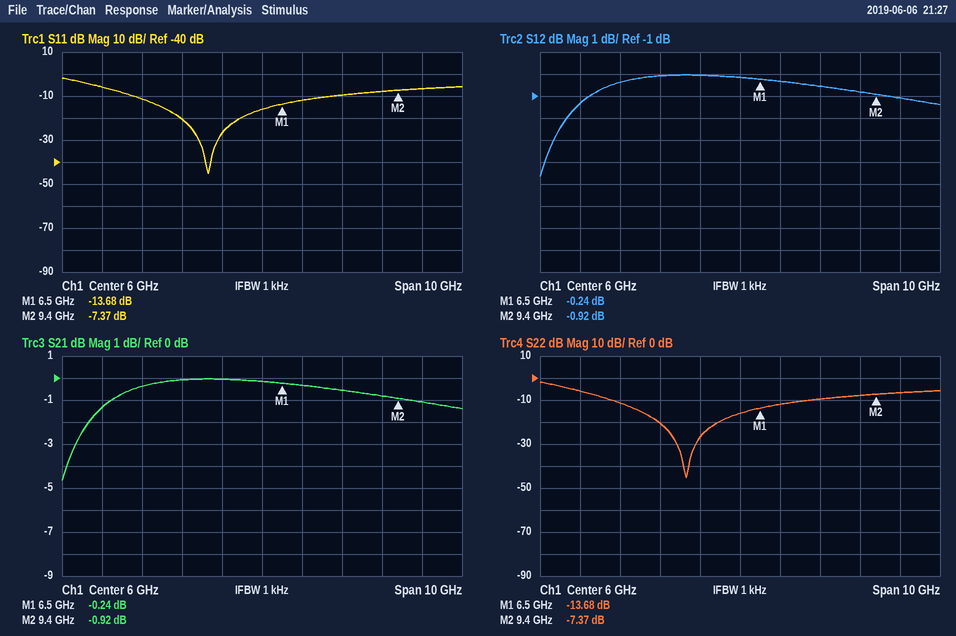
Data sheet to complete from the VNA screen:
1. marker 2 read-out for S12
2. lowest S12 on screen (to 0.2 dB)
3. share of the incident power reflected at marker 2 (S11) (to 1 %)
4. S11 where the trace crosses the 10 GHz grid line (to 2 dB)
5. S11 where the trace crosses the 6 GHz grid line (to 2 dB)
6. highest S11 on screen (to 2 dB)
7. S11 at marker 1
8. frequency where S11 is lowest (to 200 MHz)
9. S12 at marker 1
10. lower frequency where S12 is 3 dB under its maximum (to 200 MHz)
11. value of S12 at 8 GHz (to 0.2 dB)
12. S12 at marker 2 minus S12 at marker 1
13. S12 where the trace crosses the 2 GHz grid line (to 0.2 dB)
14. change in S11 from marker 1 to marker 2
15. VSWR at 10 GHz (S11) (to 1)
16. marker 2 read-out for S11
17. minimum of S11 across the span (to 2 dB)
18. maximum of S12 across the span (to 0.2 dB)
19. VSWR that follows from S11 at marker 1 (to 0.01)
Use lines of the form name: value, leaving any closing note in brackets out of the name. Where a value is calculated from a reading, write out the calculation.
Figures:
marker 2 read-out for S12: -0.92 dB
lowest S12 on screen: -4.6 dB
share of the incident power reflected at marker 2 (S11): 10^(-7.37/10) ≈ 18 %
S11 where the trace crosses the 10 GHz grid line: -6 dB
S11 where the trace crosses the 6 GHz grid line: -16 dB
highest S11 on screen: -2 dB
S11 at marker 1: -13.68 dB
frequency where S11 is lowest: 4.6 GHz
S12 at marker 1: -0.24 dB
lower frequency where S12 is 3 dB under its maximum: 1.4 GHz
value of S12 at 8 GHz: -0.6 dB
S12 at marker 2 minus S12 at marker 1: -0.92 − (-0.24) = -0.68 dB
S12 where the trace crosses the 2 GHz grid line: -1.4 dB
change in S11 from marker 1 to marker 2: -7.37 − (-13.68) = 6.31 dB
VSWR at 10 GHz (S11): |Γ| = 10^(-6/20) = 0.5012; VSWR = (1 + 0.5012)/(1 − 0.5012) ≈ 3
marker 2 read-out for S11: -7.37 dB
minimum of S11 across the span: -46 dB
maximum of S12 across the span: 0.0 dB
VSWR that follows from S11 at marker 1: (1 + 0.2070)/(1 − 0.2070) ≈ 1.52
